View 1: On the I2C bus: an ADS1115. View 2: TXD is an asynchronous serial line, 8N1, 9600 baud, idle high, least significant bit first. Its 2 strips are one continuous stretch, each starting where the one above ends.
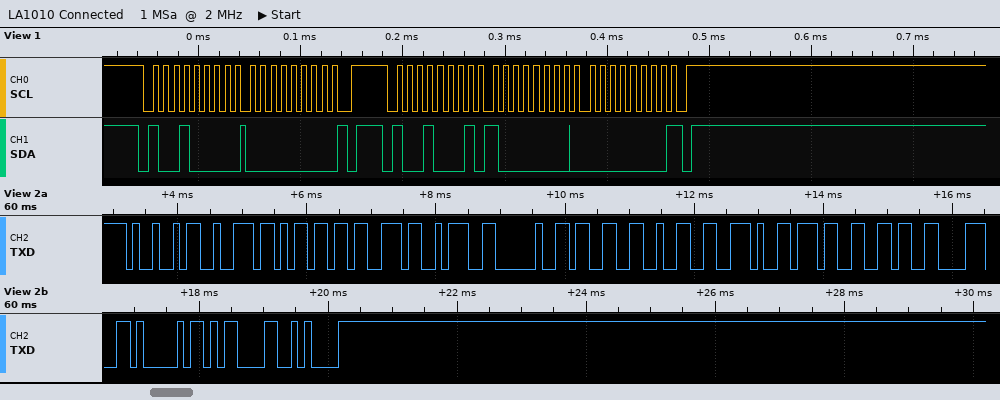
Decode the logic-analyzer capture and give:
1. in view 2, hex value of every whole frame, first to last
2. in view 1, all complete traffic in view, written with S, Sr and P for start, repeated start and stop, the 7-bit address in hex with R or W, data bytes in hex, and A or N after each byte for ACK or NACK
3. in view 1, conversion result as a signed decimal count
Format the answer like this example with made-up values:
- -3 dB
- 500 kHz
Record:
- 49 72 6D 73 3A 20 33 32 2E 37 36 38 41 0D 0A
- S 48W A 00 A P S 48R A 80 A 00 N P
- -32768
